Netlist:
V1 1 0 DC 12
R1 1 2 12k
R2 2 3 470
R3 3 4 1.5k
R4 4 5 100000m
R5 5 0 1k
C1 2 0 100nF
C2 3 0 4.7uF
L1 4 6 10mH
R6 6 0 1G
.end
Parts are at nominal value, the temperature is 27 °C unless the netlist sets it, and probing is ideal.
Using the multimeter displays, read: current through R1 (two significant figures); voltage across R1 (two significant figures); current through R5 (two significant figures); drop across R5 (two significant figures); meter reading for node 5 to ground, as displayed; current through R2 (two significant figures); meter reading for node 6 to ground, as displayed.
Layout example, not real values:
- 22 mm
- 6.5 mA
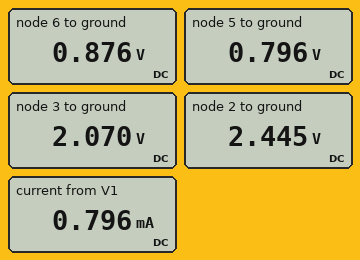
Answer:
- 800 µA
- 9.6 V
- 800 µA
- 800 mV
- 0.796 V
- 800 µA
- 0.876 V
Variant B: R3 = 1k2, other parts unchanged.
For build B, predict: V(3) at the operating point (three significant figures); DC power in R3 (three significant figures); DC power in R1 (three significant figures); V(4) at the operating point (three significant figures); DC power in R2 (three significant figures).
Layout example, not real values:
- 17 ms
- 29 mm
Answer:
- 1.87 V
- 792 µW
- 7.92 mW
- 894 mV
- 310 µW
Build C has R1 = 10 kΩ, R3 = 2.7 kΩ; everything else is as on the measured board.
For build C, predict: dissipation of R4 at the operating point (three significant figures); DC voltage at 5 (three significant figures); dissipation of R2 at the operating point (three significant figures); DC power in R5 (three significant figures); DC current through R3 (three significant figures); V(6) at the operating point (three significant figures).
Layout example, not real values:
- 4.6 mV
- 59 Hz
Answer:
- 70.7 µW
- 841 mV
- 332 µW
- 707 µW
- 841 µA
- 925 mV
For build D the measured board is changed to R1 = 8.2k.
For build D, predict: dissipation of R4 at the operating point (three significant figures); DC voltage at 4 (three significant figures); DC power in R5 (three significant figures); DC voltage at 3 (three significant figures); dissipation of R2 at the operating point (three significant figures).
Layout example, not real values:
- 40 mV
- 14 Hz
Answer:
- 113 µW
- 1.17 V
- 1.13 mW
- 2.77 V
- 533 µW
